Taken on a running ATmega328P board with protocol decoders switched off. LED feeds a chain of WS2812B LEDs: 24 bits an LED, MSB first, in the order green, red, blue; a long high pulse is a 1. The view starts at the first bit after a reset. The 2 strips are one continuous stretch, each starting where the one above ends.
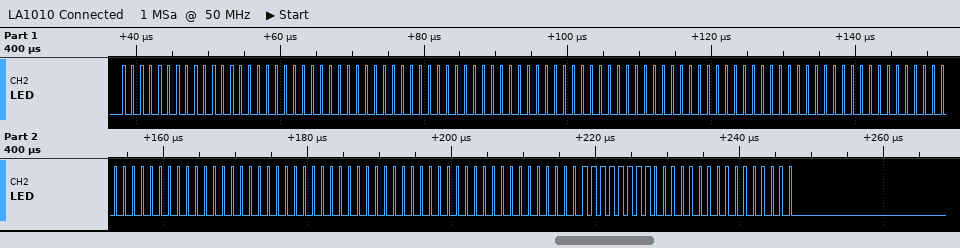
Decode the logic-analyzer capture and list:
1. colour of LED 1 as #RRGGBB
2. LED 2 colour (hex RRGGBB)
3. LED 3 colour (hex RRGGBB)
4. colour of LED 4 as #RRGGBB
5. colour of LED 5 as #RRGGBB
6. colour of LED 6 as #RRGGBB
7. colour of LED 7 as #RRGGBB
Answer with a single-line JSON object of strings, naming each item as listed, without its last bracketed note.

{"colour of LED 1 as #RRGGBB": "#000000", "LED 2 colour": "#000000", "LED 3 colour": "#000000", "colour of LED 4 as #RRGGBB": "#000000", "colour of LED 5 as #RRGGBB": "#000000", "colour of LED 6 as #RRGGBB": "#000000", "colour of LED 7 as #RRGGBB": "#00FF00"}
